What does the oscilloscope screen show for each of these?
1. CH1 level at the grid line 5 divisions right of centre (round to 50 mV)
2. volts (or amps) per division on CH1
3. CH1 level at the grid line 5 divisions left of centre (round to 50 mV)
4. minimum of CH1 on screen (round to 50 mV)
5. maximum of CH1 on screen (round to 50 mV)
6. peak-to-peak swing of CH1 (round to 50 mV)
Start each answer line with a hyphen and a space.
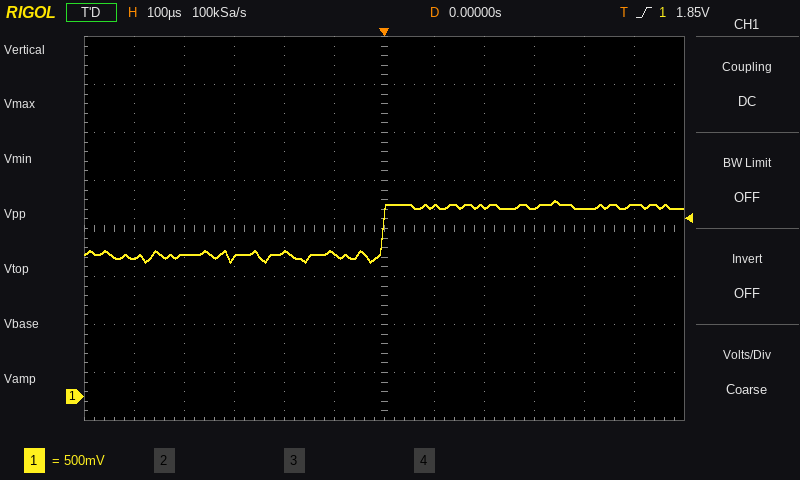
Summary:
- 2.00 V
- 500 mV
- 1.45 V
- 1.40 V
- 2.05 V
- 650 mV
